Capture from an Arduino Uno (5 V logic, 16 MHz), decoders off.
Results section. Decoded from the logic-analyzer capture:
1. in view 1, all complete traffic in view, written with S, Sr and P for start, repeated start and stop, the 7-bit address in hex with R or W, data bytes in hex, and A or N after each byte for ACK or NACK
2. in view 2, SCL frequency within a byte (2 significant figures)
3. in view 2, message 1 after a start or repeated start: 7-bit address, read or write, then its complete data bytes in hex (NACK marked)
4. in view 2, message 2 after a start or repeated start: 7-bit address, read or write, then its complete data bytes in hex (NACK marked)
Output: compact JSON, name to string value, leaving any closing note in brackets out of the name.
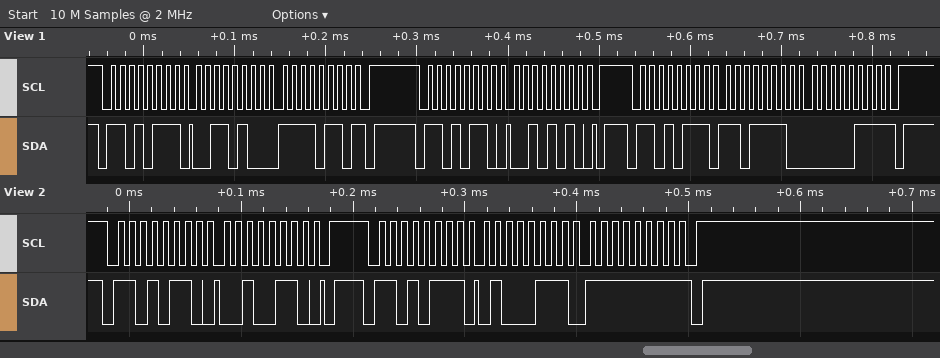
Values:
{"in view 1, all complete traffic in view, written with S, Sr and P for start, repeated start and stop, the 7-bit address in hex with R or W, data bytes in hex, and A or N after each byte for ACK or NACK": "S 6BR A 34 A F6 N P S 6BW A 2A A P S 6BR A DE A 07 N P", "in view 2, SCL frequency within a byte": "100 kHz", "in view 2, message 1 after a start or repeated start: 7-bit address, read or write, then its complete data bytes in hex": "0x6B write: 26", "in view 2, message 2 after a start or repeated start: 7-bit address, read or write, then its complete data bytes in hex": "0x6B read: 47 FF NACK"}
